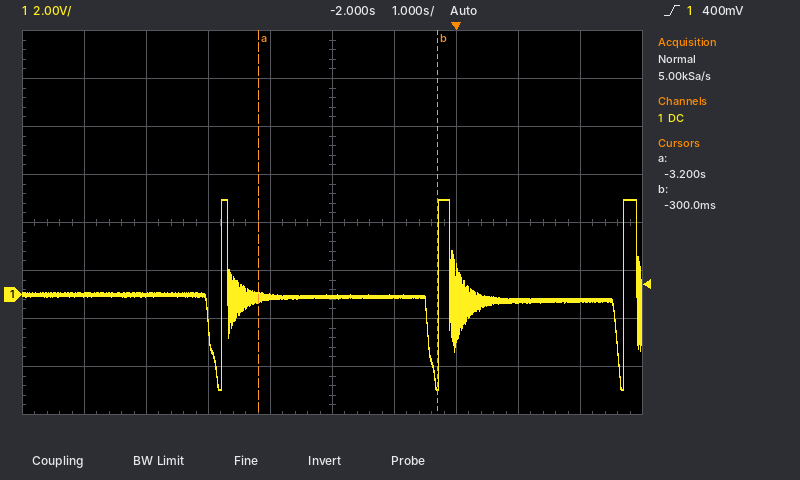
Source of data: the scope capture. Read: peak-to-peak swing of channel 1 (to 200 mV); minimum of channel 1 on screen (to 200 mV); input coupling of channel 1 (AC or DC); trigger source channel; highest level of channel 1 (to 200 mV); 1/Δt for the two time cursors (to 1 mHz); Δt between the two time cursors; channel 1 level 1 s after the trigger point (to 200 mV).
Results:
8.0 V
-4.0 V
DC
channel 1
4.0 V
345 mHz
2.9 s
-200 mV
